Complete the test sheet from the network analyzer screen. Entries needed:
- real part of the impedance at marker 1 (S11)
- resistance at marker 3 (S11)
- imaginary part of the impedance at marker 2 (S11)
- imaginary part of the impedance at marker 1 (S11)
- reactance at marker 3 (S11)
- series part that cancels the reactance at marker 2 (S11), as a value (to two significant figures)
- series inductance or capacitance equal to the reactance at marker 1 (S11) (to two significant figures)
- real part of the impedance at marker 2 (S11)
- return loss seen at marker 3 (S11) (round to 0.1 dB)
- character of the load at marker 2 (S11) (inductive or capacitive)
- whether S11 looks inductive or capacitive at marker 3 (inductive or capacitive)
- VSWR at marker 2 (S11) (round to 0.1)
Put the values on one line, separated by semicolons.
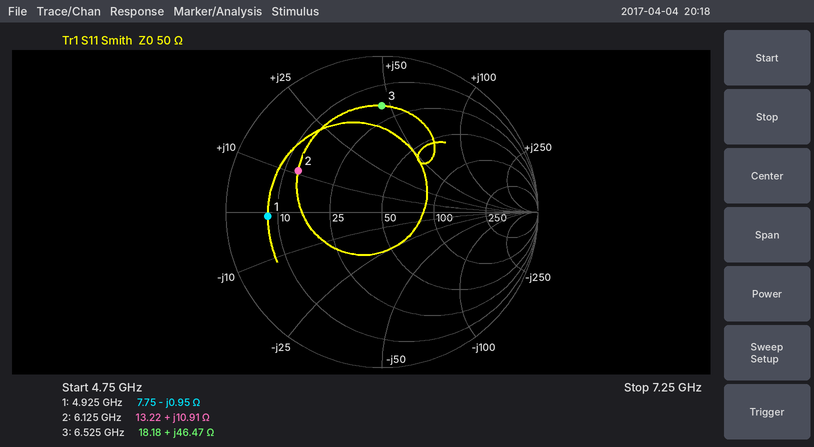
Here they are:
7.75 Ω; 18.18 Ω; +10.91 Ω; -0.95 Ω; +46.47 Ω; 2.4 pF; 34 pF; 13.22 Ω; 3.3 dB; inductive; inductive; 4.0
